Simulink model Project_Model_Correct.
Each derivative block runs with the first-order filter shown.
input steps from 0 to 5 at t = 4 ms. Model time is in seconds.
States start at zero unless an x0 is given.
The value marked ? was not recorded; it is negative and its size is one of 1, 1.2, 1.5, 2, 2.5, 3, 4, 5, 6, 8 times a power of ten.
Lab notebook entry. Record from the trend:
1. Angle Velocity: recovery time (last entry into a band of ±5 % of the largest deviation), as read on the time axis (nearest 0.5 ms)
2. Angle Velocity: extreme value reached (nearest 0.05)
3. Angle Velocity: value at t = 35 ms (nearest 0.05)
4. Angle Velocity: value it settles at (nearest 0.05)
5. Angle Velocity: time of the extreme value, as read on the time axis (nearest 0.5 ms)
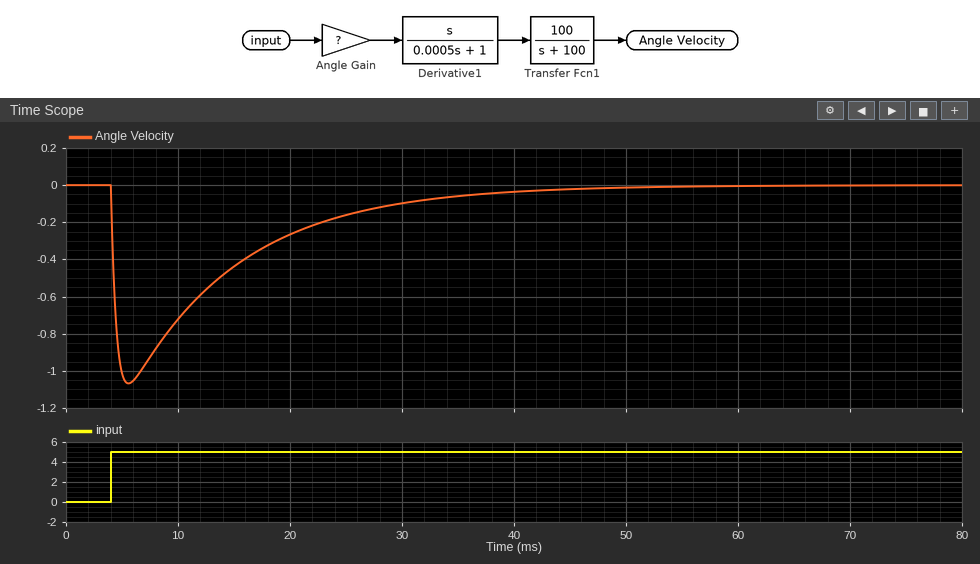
36.0 ms
-1.05
-0.05
0.00
5.5 ms
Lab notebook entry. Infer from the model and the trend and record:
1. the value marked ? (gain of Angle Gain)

-0.0025
